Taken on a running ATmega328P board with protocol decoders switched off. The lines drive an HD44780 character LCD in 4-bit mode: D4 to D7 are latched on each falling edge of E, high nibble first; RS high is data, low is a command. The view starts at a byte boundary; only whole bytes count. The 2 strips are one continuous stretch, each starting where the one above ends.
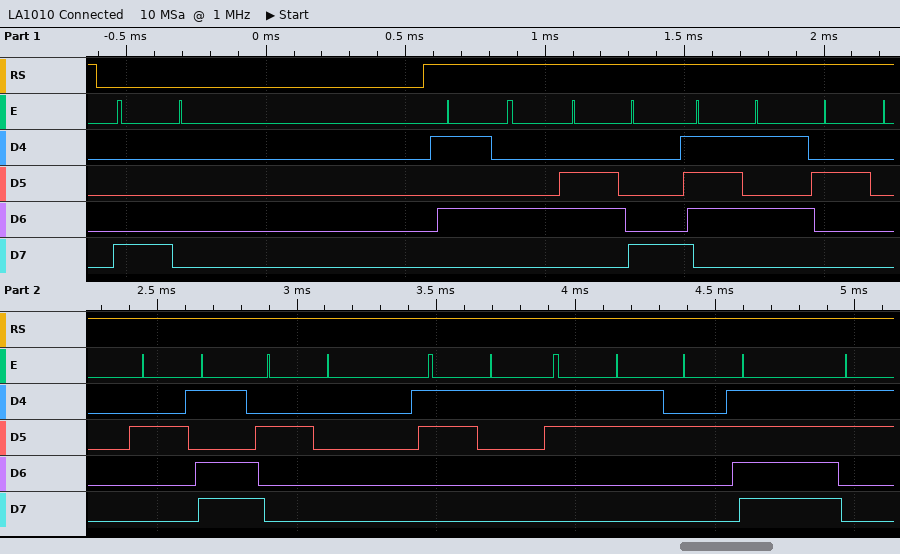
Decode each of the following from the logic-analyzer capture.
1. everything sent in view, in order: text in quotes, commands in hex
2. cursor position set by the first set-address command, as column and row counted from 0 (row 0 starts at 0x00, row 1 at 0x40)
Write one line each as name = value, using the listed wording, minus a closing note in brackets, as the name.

everything sent in view, in order: text in quotes, commands in hex = 0x80 "Thu - 13/"
cursor position set by the first set-address command, as column and row counted from 0 = column 0, row 0
